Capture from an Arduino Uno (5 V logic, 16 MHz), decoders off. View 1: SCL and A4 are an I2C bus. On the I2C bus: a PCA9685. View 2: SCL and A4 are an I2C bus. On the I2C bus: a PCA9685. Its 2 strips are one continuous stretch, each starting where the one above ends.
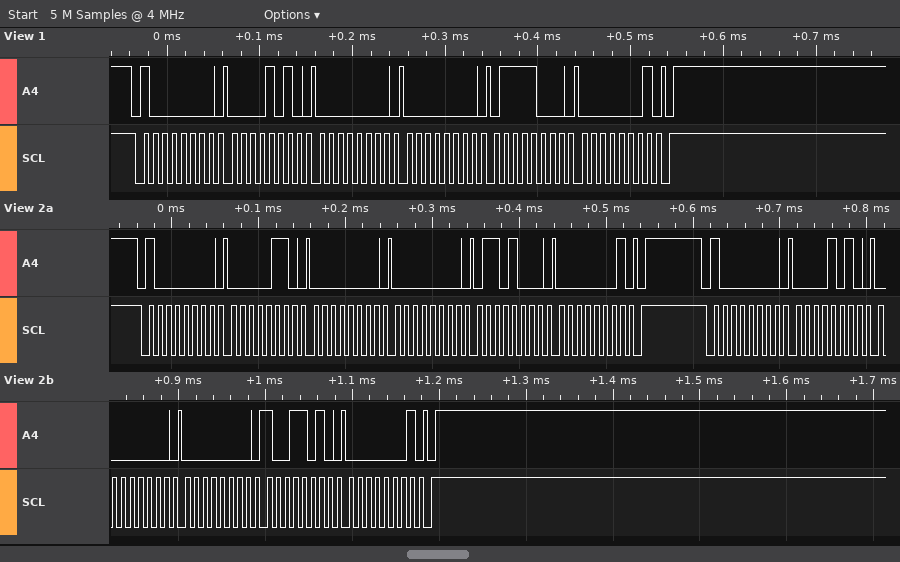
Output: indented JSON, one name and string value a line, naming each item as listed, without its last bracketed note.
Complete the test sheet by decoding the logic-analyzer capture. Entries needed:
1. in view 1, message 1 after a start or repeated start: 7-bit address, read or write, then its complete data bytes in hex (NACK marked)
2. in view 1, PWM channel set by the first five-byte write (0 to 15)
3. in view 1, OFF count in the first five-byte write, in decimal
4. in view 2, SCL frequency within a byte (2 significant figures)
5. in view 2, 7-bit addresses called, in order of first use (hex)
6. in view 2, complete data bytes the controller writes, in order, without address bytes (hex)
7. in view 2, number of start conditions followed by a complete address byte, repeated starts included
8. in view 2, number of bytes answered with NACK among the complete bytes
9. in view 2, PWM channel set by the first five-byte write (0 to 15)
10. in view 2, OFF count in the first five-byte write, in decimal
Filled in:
{
  "in view 1, message 1 after a start or repeated start: 7-bit address, read or write, then its complete data bytes in hex": "0x40 write: 0A 00 00 78 01",
  "in view 1, PWM channel set by the first five-byte write": "1",
  "in view 1, OFF count in the first five-byte write, in decimal": "376",
  "in view 2, SCL frequency within a byte": "100 kHz",
  "in view 2, 7-bit addresses called, in order of first use": "0x40",
  "in view 2, complete data bytes the controller writes, in order, without address bytes": "06 00 00 68 01 0A 00 00 9A 01",
  "in view 2, number of start conditions followed by a complete address byte, repeated starts included": "2",
  "in view 2, number of bytes answered with NACK among the complete bytes": "0",
  "in view 2, PWM channel set by the first five-byte write": "0",
  "in view 2, OFF count in the first five-byte write, in decimal": "360"
}
